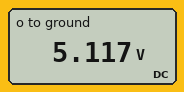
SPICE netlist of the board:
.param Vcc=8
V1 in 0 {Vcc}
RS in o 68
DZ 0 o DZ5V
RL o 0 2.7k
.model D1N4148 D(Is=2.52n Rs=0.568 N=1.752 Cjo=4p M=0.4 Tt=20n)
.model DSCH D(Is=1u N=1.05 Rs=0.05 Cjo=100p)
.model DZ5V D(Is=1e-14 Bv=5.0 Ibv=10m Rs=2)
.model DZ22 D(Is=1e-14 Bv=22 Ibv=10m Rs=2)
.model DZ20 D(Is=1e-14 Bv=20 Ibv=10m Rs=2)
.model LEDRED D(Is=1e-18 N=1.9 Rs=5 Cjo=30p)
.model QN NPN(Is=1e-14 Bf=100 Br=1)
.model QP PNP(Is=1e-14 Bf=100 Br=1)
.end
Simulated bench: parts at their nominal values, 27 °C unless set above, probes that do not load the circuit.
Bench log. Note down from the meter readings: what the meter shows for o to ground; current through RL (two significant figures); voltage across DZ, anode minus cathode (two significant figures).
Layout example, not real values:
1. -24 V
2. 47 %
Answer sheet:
1. 5.117 V
2. 1.9 mA
3. -5.1 V
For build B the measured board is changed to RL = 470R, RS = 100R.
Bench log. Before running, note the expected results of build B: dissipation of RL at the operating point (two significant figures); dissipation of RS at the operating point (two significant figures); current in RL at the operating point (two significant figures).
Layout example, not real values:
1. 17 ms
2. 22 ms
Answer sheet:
1. 54 mW
2. 87 mW
3. 11 mA
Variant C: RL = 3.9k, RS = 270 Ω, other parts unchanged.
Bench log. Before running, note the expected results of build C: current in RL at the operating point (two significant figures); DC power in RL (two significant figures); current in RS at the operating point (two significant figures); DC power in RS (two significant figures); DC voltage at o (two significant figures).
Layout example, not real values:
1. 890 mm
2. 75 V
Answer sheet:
1. 1.3 mA
2. 6.5 mW
3. 11 mA
4. 33 mW
5. 5.0 V
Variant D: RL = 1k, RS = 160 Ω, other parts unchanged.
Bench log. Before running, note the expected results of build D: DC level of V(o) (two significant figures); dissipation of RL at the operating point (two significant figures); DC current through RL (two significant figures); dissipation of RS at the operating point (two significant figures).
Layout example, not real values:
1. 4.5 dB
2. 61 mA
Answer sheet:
1. 5.0 V
2. 25 mW
3. 5.0 mA
4. 55 mW
